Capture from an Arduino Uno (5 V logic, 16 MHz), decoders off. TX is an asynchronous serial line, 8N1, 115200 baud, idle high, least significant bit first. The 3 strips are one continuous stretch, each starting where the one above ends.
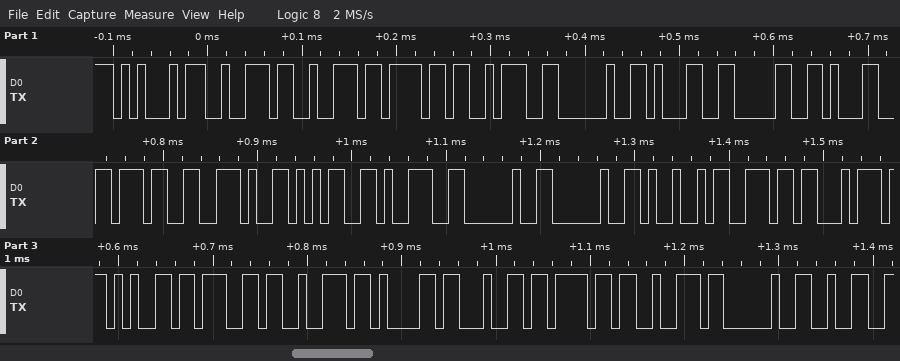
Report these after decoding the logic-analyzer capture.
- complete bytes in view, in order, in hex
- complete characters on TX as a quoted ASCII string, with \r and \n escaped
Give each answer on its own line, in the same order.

45 72 72 6F 3A 20 31 30 31 37 2E 35 39 20 20 49 6E 74 65 67 72 61 64 6F 72 20 32
"Erro: 1017.59  Integrador 2"
